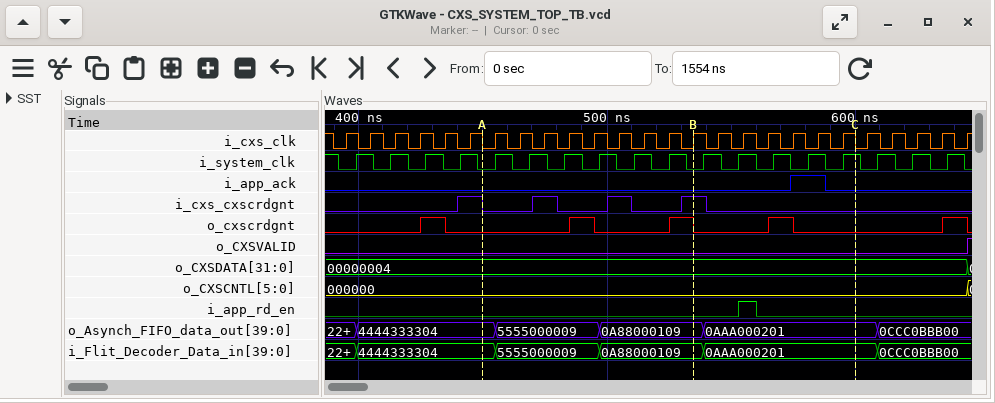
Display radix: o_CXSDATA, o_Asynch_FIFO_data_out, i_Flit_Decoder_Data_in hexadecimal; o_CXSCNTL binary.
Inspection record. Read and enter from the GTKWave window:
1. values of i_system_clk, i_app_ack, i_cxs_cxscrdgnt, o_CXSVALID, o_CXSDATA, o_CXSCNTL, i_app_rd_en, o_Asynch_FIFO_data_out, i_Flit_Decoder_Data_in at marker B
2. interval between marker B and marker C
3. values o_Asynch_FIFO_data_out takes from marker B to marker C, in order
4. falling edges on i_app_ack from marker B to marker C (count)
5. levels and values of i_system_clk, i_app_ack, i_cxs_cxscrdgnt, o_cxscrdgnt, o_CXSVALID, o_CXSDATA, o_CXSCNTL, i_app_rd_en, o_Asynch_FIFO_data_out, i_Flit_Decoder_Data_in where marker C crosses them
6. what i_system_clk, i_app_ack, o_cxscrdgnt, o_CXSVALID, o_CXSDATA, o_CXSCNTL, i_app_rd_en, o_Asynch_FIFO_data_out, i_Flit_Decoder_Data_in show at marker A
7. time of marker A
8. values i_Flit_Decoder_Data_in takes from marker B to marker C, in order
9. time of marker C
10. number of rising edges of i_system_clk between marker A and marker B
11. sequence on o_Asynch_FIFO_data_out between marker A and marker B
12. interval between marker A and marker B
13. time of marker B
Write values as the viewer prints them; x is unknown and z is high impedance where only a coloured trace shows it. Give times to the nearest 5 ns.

i_system_clk=0, i_app_ack=0, i_cxs_cxscrdgnt=1, o_CXSVALID=0, o_CXSDATA=00000004, o_CXSCNTL=000000, i_app_rd_en=0, o_Asynch_FIFO_data_out=0A88000109, i_Flit_Decoder_Data_in=0A88000109
65 ns
0A88000109, 0AAA000201
1
i_system_clk=1, i_app_ack=0, i_cxs_cxscrdgnt=0, o_cxscrdgnt=0, o_CXSVALID=0, o_CXSDATA=00000004, o_CXSCNTL=000000, i_app_rd_en=0, o_Asynch_FIFO_data_out=0AAA000201, i_Flit_Decoder_Data_in=0AAA000201
i_system_clk=0, i_app_ack=0, o_cxscrdgnt=0, o_CXSVALID=0, o_CXSDATA=00000004, o_CXSCNTL=000000, i_app_rd_en=0, o_Asynch_FIFO_data_out=4444333304, i_Flit_Decoder_Data_in=4444333304
450 ns
0A88000109, 0AAA000201
600 ns
6
4444333304, 5555000009, 0A88000109
85 ns
535 ns
